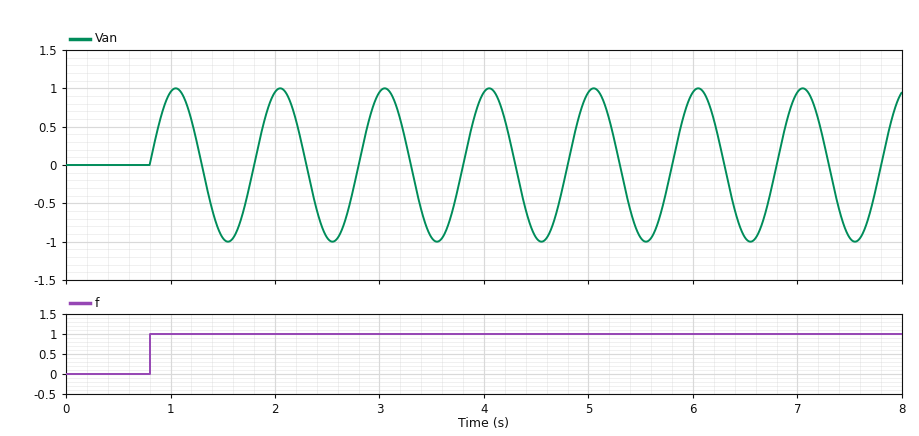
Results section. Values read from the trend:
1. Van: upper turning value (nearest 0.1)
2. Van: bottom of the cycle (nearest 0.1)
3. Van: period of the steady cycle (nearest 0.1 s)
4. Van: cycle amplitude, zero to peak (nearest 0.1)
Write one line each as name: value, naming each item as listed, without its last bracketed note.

Van: upper turning value: 1.0
Van: bottom of the cycle: -1.0
Van: period of the steady cycle: 1.0 s
Van: cycle amplitude, zero to peak: 1.0
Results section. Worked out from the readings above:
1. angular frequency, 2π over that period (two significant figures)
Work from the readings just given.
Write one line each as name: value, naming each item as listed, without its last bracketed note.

angular frequency, 2π over that period: 6.3 rad/s
